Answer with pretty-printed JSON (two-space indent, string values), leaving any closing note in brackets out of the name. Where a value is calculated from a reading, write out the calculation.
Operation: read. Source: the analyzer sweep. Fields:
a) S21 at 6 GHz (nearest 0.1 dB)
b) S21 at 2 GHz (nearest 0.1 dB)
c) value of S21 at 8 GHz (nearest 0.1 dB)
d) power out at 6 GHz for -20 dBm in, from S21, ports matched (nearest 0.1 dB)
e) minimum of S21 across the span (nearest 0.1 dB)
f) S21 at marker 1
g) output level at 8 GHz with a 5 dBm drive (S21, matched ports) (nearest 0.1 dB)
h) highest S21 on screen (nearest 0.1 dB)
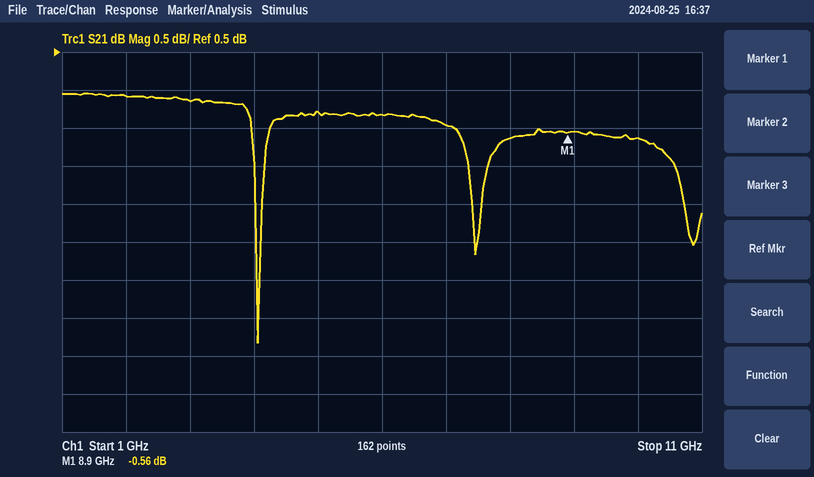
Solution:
{
  "S21 at 6 GHz": "-0.3 dB",
  "S21 at 2 GHz": "-0.1 dB",
  "value of S21 at 8 GHz": "-0.6 dB",
  "power out at 6 GHz for -20 dBm in, from S21, ports matched": "-20 dBm + (-0.3 dB) = -20.3 dBm",
  "minimum of S21 across the span": "-3.3 dB",
  "S21 at marker 1": "-0.56 dB",
  "output level at 8 GHz with a 5 dBm drive (S21, matched ports)": "5 dBm + (-0.6 dB) = 4.4 dBm",
  "highest S21 on screen": "0.0 dB"
}
